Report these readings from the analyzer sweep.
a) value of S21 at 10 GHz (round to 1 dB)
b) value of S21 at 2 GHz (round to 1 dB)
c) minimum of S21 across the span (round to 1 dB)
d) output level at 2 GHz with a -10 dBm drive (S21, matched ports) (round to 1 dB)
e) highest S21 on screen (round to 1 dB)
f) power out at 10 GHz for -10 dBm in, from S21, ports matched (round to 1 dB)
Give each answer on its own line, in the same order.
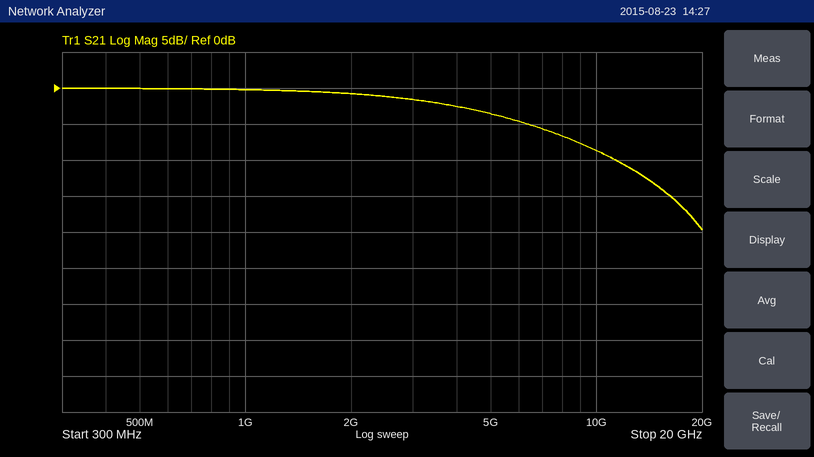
-9 dB
-1 dB
-20 dB
-11 dBm
0 dB
-19 dBm
